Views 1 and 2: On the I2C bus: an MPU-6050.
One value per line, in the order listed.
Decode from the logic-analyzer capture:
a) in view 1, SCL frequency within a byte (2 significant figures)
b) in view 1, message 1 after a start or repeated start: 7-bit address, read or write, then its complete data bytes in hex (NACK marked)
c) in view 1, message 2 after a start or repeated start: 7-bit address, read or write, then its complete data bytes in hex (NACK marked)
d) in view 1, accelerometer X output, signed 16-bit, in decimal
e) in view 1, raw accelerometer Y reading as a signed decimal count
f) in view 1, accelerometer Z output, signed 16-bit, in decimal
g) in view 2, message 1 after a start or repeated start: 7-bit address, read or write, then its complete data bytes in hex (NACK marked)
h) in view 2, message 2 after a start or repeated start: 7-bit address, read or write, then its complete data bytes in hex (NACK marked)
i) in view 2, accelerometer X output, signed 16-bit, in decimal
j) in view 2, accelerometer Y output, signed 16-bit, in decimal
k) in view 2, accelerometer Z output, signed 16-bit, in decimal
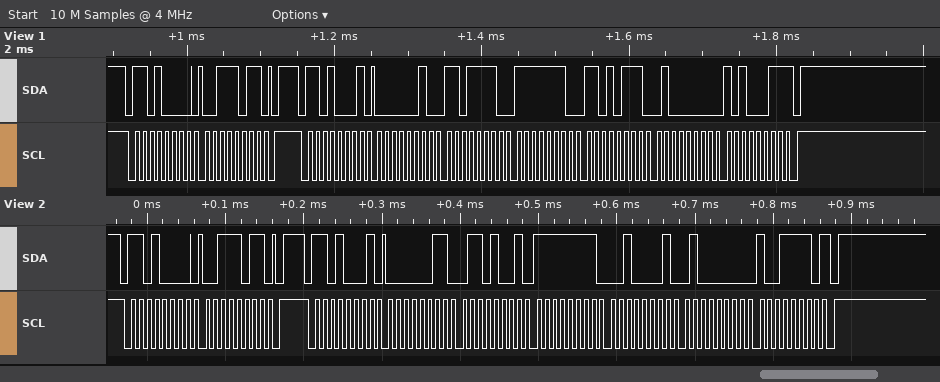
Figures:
100 kHz
0x68 write: 3B
0x68 read: 02 DE FE D7 40 A3 NACK
734
-297
16547
0x68 write: 3B
0x68 read: 03 69 FF 21 40 9E NACK
873
-223
16542
